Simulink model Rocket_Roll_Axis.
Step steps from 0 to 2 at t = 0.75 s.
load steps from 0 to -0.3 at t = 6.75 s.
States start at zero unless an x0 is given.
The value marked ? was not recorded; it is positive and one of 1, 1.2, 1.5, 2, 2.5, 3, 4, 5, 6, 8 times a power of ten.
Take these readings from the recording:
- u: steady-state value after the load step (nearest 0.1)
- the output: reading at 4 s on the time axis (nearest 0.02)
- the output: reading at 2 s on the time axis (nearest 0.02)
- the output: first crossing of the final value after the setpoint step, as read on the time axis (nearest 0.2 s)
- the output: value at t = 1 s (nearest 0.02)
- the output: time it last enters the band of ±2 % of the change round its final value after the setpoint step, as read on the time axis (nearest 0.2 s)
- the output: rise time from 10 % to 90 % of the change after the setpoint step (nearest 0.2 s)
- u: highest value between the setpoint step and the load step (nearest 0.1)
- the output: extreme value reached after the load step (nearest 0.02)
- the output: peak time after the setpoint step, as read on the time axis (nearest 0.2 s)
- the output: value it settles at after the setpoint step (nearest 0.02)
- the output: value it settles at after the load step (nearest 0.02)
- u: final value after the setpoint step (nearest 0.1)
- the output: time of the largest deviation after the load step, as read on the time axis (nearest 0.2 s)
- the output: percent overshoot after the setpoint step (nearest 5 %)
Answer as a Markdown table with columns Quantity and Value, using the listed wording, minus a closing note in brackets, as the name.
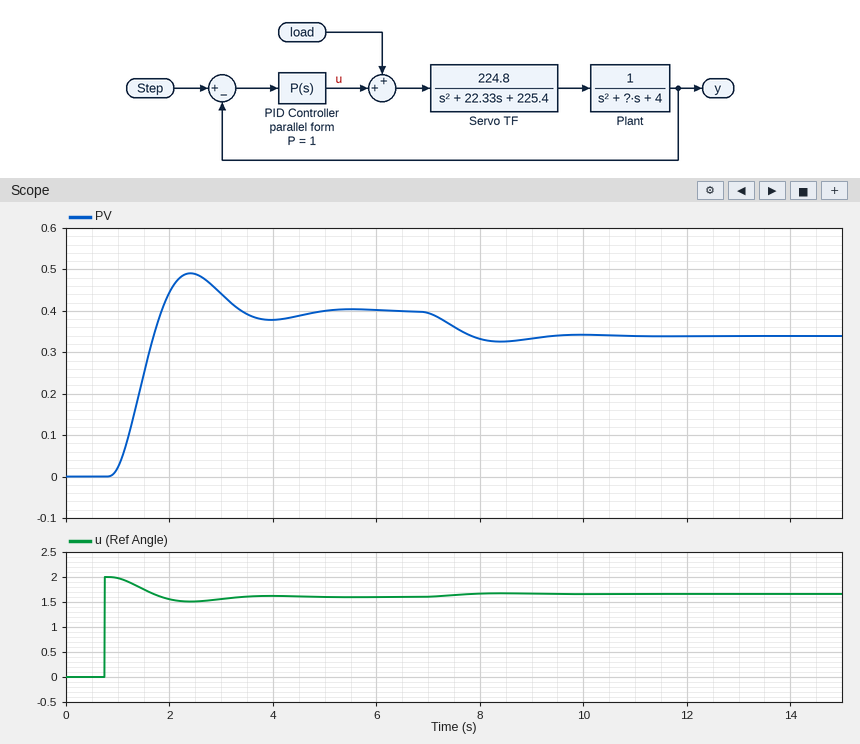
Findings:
| Quantity | Value |
|---|---|
| u: steady-state value after the load step | 1.7 |
| the output: reading at 4 s on the time axis | 0.38 |
| the output: reading at 2 s on the time axis | 0.44 |
| the output: first crossing of the final value after the setpoint step, as read on the time axis | 1.8 s |
| the output: value at t = 1 s | 0.02 |
| the output: time it last enters the band of ±2 % of the change round its final value after the setpoint step, as read on the time axis | 4.6 s |
| the output: rise time from 10 % to 90 % of the change after the setpoint step | 0.6 s |
| u: highest value between the setpoint step and the load step | 2.0 |
| the output: extreme value reached after the load step | 0.32 |
| the output: peak time after the setpoint step, as read on the time axis | 2.4 s |
| the output: value it settles at after the setpoint step | 0.40 |
| the output: value it settles at after the load step | 0.34 |
| u: final value after the setpoint step | 1.6 |
| the output: time of the largest deviation after the load step, as read on the time axis | 8.4 s |
| the output: percent overshoot after the setpoint step | 25 % |
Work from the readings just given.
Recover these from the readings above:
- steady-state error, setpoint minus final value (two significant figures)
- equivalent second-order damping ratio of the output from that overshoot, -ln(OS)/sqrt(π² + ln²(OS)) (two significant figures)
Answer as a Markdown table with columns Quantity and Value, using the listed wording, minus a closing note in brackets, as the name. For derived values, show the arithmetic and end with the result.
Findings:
| Quantity | Value |
|---|---|
| steady-state error, setpoint minus final value | 2 - 0.4 = 1.6 |
| equivalent second-order damping ratio of the output from that overshoot, -ln(OS)/sqrt(π² + ln²(OS)) | ln(0.25) = -1.386; 1.386 / sqrt(9.870 + 1.922) = 0.40 |
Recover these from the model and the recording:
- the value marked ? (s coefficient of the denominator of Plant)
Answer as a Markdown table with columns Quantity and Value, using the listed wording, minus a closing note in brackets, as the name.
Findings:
| Quantity | Value |
|---|---|
| the value marked ? | 2 |
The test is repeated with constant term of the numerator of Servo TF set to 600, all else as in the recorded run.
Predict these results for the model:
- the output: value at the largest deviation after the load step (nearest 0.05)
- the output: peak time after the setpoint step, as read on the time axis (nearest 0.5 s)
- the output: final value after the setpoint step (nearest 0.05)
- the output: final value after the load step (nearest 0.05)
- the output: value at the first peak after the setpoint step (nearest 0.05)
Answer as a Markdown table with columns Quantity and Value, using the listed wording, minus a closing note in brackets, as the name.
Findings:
| Quantity | Value |
|---|---|
| the output: value at the largest deviation after the load step | 0.65 |
| the output: peak time after the setpoint step, as read on the time axis | 2.0 s |
| the output: final value after the setpoint step | 0.80 |
| the output: final value after the load step | 0.70 |
| the output: value at the first peak after the setpoint step | 1.05 |
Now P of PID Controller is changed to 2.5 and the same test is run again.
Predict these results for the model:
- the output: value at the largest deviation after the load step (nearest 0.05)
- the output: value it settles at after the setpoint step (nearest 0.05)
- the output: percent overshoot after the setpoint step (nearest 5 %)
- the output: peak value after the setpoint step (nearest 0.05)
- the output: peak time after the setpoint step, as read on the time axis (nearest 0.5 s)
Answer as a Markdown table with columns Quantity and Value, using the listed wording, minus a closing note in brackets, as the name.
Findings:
| Quantity | Value |
|---|---|
| the output: value at the largest deviation after the load step | 0.70 |
| the output: value it settles at after the setpoint step | 0.75 |
| the output: percent overshoot after the setpoint step | 30 % |
| the output: peak value after the setpoint step | 1.00 |
| the output: peak time after the setpoint step, as read on the time axis | 2.0 s |
